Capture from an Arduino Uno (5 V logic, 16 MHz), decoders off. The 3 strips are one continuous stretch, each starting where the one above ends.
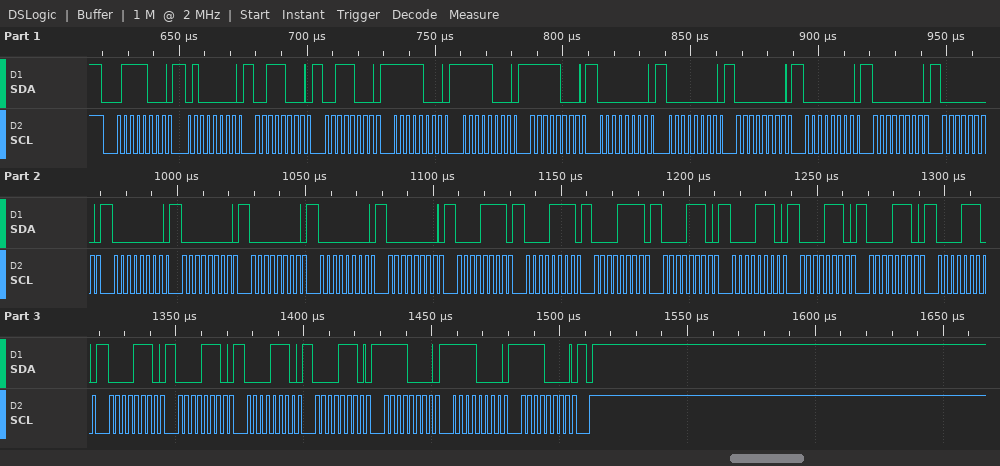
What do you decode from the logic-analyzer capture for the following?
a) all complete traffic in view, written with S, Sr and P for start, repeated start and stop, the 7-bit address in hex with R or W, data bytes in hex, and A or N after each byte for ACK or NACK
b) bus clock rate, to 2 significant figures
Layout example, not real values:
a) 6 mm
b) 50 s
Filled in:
a) S 3CW A 40 A 38 A 38 A F8 A F8 A F8 A 00 A 00 A 00 A 00 A 00 A 00 A 00 A 00 A 00 A 00 A 00 A 0F A 0F A 0F A 0E A 0E A 0E A 0E A 0E A 0E A 0E A 0E A 0E A F0 A F0 A F0 A P
b) 400 kHz
